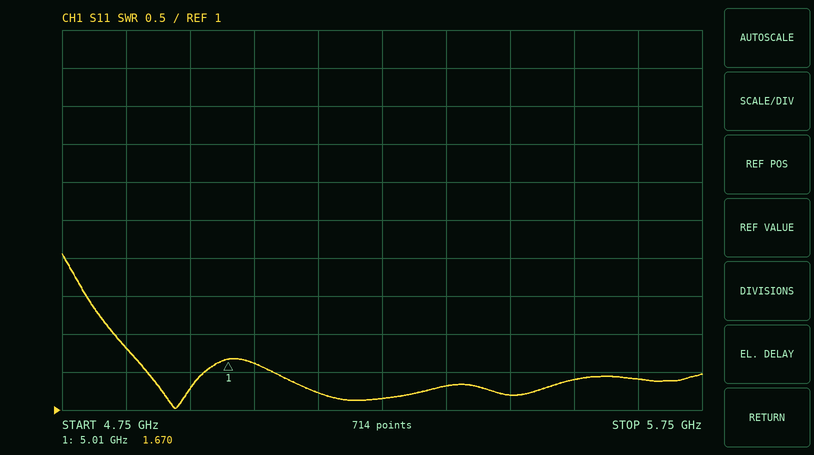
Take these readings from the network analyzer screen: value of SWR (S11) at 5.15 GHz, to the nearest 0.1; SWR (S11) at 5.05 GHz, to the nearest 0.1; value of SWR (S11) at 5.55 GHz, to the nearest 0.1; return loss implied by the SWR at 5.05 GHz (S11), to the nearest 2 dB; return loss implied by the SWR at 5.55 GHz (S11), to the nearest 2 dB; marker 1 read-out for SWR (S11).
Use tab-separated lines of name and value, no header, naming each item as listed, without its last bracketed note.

value of SWR (S11) at 5.15 GHz, to the nearest 0.1	1.2
SWR (S11) at 5.05 GHz, to the nearest 0.1	1.6
value of SWR (S11) at 5.55 GHz, to the nearest 0.1	1.4
return loss implied by the SWR at 5.05 GHz (S11), to the nearest 2 dB	12 dB
return loss implied by the SWR at 5.55 GHz (S11), to the nearest 2 dB	16 dB
marker 1 read-out for SWR	1.670
